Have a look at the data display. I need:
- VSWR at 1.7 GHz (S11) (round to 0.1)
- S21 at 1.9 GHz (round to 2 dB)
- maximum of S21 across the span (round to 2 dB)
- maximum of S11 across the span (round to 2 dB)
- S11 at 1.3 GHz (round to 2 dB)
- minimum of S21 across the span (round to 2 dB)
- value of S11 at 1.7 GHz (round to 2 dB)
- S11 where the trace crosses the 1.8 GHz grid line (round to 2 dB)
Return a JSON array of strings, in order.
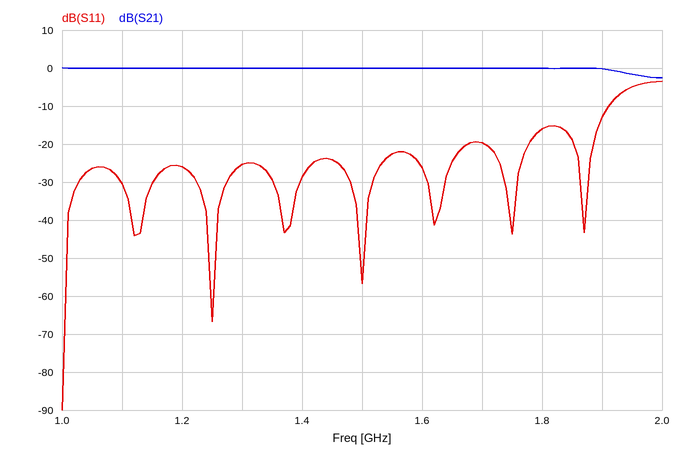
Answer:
["1.2", "0 dB", "0 dB", "-4 dB", "-26 dB", "-2 dB", "-20 dB", "-16 dB"]
